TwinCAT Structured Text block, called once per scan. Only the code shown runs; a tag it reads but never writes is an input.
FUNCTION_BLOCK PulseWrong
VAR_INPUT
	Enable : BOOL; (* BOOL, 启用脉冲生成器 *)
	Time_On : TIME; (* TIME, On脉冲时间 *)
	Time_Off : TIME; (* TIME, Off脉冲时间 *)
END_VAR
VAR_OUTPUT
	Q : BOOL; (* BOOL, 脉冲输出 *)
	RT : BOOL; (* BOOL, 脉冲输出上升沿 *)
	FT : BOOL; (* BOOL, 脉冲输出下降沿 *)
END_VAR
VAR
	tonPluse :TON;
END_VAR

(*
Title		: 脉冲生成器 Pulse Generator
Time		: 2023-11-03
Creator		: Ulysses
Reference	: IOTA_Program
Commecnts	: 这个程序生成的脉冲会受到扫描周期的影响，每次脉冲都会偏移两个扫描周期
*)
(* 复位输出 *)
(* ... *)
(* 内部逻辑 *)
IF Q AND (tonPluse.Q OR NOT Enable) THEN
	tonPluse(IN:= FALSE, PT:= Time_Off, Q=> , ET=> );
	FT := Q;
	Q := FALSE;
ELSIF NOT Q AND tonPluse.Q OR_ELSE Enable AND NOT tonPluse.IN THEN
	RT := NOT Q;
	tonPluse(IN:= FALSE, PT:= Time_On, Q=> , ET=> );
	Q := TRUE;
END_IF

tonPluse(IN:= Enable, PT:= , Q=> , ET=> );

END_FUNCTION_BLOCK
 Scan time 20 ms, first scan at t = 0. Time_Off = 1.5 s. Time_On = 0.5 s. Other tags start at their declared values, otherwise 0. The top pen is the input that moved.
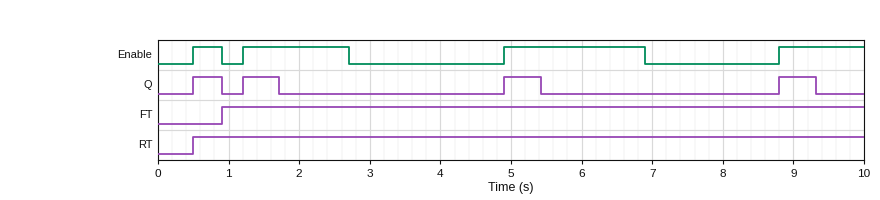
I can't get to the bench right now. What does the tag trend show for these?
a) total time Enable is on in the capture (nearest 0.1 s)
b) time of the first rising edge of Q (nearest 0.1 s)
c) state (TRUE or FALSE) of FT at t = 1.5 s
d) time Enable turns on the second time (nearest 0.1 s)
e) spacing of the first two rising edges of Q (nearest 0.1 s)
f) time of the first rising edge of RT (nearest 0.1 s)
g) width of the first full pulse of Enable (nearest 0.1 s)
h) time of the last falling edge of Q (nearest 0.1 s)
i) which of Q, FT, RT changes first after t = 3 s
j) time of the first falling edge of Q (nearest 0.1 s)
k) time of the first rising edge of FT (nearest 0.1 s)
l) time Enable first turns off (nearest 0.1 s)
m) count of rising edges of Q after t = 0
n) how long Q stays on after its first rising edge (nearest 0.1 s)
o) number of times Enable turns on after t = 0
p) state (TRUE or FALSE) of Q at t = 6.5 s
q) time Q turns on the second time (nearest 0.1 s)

5.1 s
0.5 s
TRUE
1.2 s
0.7 s
0.5 s
0.4 s
9.3 s
Q
0.9 s
0.9 s
0.9 s
4
0.4 s
4
FALSE
1.2 s
